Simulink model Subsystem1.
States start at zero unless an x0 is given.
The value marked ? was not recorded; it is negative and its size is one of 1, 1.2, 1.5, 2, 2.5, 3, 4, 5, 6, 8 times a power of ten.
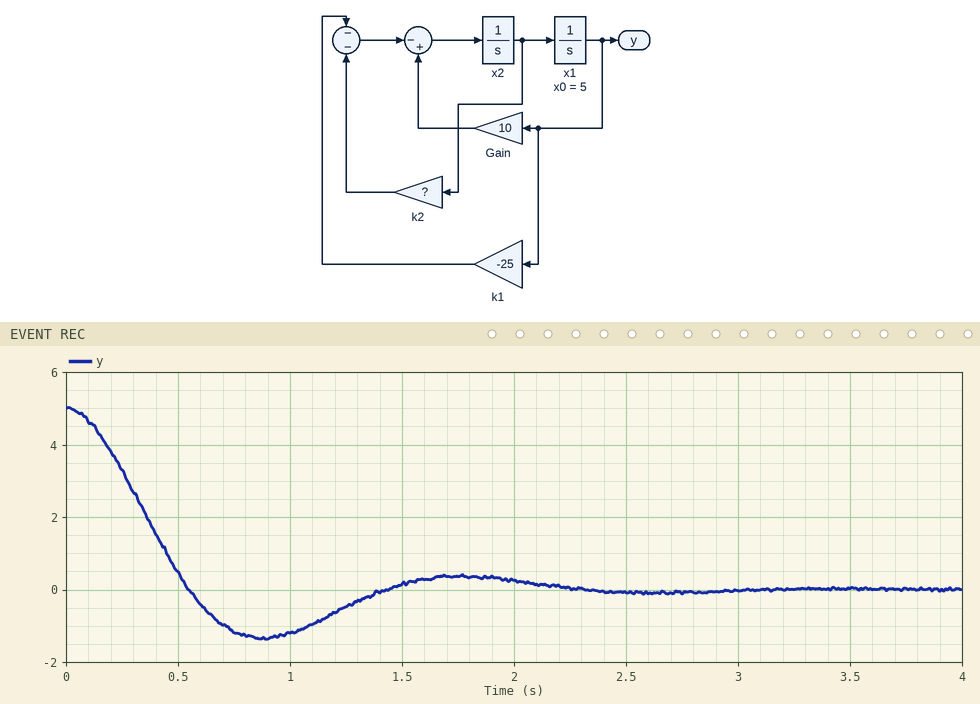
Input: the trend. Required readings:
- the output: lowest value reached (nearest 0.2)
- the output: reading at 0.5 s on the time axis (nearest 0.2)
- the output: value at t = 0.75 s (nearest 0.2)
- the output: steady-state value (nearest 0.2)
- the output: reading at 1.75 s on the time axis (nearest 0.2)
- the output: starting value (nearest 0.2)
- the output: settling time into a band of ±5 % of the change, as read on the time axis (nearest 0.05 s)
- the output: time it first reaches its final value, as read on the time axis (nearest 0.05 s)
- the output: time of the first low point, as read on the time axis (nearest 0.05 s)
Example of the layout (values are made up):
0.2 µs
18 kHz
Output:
-1.4
0.4
-1.2
0.0
0.4
5.0
2.00 s
0.55 s
0.90 s
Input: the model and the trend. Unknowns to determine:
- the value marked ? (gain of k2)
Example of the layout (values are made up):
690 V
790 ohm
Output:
-3
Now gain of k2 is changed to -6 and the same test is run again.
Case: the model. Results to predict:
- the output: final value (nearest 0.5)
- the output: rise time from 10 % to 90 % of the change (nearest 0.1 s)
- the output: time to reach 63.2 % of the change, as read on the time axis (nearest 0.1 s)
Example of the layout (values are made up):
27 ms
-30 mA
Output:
0.0
0.6 s
0.5 s
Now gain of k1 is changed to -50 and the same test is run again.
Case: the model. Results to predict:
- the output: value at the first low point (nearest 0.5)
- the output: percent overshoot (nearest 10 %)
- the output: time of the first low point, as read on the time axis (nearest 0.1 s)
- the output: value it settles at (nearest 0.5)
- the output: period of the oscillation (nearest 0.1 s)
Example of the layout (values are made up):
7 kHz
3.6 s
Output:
-2.5
50 %
0.5 s
0.0
1.0 s
